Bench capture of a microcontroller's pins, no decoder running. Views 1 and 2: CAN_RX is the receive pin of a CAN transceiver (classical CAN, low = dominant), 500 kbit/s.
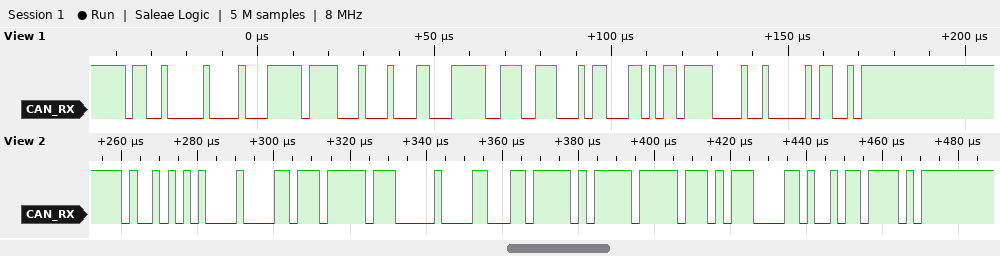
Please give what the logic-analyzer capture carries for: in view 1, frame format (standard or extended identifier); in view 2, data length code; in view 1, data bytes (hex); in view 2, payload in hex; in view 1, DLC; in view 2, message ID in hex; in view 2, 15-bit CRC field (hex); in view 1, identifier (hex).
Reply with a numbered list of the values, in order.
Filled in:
1. standard
2. 8
3. FF 88 8C 7D CE 2C 6B 78
4. 6E FF 00 63 7E FF FA E1
5. 8
6. 0x4AA
7. 0x52DE
8. 0x640
